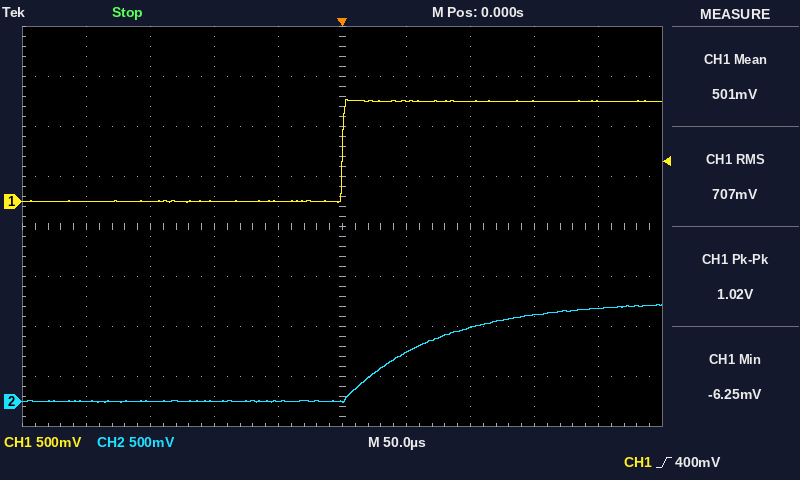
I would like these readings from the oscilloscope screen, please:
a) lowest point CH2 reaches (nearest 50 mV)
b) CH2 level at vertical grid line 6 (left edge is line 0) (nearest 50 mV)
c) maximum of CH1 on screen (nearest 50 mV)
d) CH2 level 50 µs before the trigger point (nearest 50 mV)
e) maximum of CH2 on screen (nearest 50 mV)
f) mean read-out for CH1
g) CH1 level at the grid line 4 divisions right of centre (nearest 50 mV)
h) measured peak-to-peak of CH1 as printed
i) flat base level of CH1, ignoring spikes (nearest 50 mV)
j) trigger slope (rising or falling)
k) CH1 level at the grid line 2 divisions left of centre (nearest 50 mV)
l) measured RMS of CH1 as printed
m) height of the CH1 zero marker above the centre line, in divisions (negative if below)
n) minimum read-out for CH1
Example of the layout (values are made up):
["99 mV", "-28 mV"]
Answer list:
["0 mV", "500 mV", "1.00 V", "0 mV", "950 mV", "501 mV", "1.00 V", "1.02 V", "0 mV", "rising", "0 mV", "707 mV", "+0.5 div", "-6.25 mV"]
